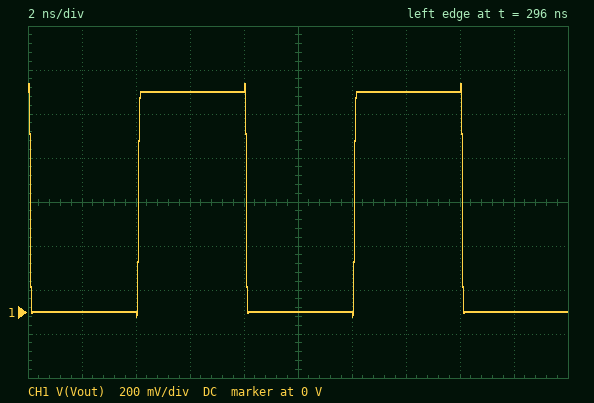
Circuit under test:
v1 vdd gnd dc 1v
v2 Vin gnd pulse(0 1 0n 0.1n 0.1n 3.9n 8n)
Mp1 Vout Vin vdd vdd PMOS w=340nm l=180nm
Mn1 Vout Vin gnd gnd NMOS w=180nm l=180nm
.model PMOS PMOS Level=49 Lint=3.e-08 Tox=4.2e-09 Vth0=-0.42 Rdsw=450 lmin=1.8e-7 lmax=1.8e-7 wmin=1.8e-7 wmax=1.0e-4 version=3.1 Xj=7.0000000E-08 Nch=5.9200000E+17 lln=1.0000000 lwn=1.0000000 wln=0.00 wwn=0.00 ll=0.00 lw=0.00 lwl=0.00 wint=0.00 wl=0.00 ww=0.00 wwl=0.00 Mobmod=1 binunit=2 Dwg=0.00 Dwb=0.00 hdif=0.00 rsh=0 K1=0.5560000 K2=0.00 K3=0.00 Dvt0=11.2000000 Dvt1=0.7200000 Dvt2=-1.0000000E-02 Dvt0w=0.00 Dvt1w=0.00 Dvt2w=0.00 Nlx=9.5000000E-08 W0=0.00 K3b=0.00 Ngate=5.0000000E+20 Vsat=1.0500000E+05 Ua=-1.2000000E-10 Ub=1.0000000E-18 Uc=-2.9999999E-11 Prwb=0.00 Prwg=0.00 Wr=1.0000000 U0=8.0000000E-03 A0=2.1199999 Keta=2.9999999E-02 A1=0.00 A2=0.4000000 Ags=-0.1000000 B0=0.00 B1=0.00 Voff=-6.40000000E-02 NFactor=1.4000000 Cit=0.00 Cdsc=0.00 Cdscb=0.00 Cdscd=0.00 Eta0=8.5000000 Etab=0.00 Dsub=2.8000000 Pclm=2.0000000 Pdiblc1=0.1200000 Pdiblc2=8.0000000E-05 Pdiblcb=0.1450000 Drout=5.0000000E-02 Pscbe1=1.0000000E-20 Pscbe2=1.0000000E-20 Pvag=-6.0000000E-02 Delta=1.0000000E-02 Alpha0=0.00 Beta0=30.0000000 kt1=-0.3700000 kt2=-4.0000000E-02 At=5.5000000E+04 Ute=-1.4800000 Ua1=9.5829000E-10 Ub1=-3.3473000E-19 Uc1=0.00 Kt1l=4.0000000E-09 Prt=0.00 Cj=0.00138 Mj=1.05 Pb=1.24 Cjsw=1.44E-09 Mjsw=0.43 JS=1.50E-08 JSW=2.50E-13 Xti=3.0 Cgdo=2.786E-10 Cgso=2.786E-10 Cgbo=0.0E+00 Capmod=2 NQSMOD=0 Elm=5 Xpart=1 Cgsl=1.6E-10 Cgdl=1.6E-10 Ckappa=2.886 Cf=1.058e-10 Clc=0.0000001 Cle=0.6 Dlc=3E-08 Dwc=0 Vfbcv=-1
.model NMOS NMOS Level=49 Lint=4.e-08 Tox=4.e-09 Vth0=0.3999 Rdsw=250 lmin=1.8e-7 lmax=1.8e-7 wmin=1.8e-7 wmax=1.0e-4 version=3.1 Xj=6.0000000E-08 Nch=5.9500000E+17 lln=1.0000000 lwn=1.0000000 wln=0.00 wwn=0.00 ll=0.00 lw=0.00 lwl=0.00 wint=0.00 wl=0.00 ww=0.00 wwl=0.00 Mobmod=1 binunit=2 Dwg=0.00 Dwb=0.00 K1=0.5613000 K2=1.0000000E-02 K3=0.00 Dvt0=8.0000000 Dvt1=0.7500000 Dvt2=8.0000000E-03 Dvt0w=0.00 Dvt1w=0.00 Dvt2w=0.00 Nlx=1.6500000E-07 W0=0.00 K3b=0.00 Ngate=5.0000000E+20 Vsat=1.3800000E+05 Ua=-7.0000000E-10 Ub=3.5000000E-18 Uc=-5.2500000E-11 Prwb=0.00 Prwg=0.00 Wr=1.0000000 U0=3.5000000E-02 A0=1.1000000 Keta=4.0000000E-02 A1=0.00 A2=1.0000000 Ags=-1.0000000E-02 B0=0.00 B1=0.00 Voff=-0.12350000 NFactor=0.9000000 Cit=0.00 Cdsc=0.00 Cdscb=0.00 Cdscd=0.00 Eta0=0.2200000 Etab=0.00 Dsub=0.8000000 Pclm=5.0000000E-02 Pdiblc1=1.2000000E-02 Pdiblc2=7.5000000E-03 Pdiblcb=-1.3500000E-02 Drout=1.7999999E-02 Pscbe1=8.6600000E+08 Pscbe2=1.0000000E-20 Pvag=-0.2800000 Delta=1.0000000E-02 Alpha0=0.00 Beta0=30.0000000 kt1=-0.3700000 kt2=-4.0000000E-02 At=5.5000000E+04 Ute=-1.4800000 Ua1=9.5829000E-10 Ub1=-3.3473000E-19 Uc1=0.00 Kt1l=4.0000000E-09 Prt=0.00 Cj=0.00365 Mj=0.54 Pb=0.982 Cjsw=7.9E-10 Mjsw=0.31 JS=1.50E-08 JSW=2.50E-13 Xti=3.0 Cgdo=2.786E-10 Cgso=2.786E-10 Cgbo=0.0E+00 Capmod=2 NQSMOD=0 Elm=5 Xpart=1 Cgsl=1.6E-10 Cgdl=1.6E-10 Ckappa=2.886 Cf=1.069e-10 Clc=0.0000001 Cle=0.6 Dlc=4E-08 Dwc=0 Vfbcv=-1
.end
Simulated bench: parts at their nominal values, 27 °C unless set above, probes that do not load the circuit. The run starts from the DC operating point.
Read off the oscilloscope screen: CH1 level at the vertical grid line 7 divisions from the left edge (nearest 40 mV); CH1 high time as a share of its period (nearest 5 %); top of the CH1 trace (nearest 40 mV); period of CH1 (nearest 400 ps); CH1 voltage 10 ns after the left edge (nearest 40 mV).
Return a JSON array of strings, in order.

["1.00 V", "50 %", "1.04 V", "8.0 ns", "0 V"]
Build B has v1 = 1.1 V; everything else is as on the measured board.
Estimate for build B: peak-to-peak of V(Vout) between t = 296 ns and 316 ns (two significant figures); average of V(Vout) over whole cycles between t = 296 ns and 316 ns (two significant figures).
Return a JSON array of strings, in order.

["1.2 V", "550 mV"]
